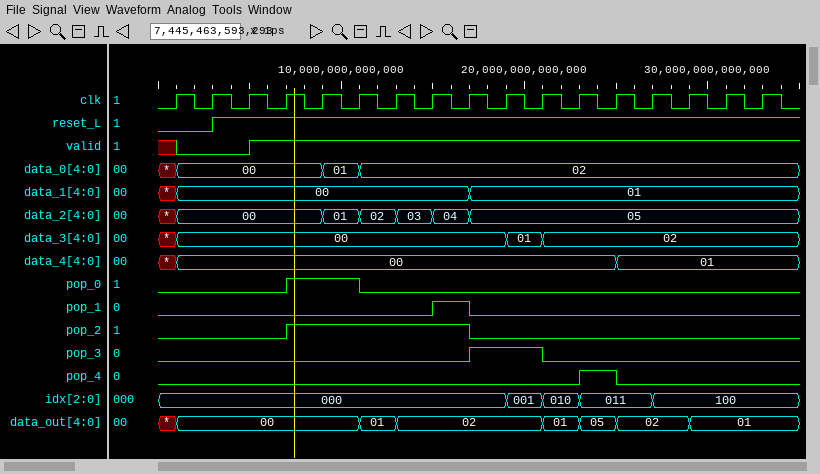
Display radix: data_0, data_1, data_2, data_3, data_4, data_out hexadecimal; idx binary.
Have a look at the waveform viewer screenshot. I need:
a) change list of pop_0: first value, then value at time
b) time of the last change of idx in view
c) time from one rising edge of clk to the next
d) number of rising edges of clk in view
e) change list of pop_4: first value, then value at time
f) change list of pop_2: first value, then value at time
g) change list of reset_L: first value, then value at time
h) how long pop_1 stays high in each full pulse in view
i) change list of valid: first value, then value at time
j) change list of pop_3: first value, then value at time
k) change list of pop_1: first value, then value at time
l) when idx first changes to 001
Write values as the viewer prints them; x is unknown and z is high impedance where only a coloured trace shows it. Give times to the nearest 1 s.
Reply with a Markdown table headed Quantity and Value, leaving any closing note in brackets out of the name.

| Quantity | Value |
|---|---|
| change list of pop_0: first value, then value at time | 0, 1 at 7 s, 0 at 11 s |
| time of the last change of idx in view | 27 s |
| time from one rising edge of clk to the next | 2 s |
| number of rising edges of clk in view | 17 |
| change list of pop_4: first value, then value at time | 0, 1 at 23 s, 0 at 25 s |
| change list of pop_2: first value, then value at time | 0, 1 at 7 s, 0 at 17 s |
| change list of reset_L: first value, then value at time | 0, 1 at 3 s |
| how long pop_1 stays high in each full pulse in view | 2 s |
| change list of valid: first value, then value at time | x, 0 at 1 s, 1 at 5 s |
| change list of pop_3: first value, then value at time | 0, 1 at 17 s, 0 at 21 s |
| change list of pop_1: first value, then value at time | 0, 1 at 15 s, 0 at 17 s |
| when idx first changes to 001 | 19 s |
